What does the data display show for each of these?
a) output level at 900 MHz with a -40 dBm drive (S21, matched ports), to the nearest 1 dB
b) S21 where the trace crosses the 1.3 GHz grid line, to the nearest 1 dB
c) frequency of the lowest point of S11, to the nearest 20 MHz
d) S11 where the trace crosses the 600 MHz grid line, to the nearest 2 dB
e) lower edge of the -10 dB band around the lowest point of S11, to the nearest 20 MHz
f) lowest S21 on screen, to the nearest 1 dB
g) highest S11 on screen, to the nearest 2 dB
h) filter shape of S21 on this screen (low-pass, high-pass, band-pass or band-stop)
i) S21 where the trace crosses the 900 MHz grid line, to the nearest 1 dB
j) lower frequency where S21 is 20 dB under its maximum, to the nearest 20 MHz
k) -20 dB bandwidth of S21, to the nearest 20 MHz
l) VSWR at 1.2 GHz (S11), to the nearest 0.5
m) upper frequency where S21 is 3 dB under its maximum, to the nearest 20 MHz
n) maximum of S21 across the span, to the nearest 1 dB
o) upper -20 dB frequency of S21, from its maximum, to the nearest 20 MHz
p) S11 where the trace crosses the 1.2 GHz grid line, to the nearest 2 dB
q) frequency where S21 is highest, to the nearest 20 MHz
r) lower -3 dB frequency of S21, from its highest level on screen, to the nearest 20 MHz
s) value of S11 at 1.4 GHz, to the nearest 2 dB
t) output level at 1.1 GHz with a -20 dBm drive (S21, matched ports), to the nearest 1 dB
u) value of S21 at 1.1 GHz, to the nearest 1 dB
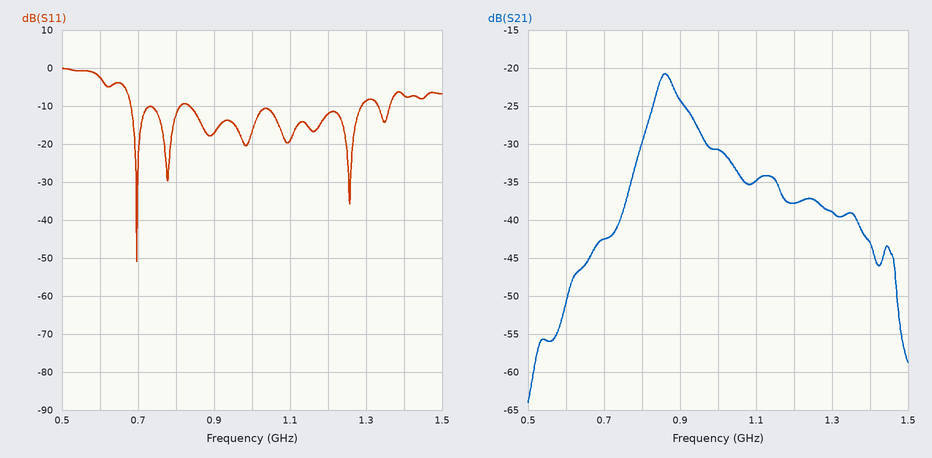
-64 dBm
-39 dB
700 MHz
-2 dB
680 MHz
-64 dB
0 dB
band-pass
-24 dB
740 MHz
640 MHz
1.5
900 MHz
-21 dB
1.38 GHz
-12 dB
860 MHz
840 MHz
-8 dB
-55 dBm
-35 dB
